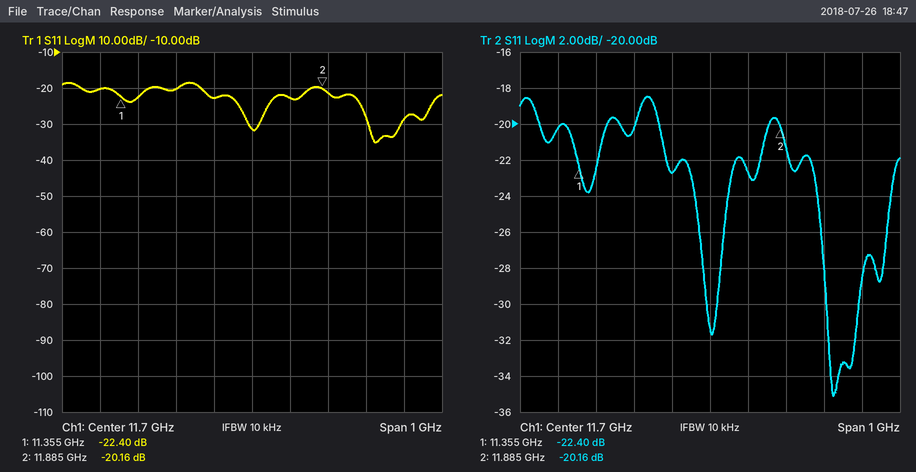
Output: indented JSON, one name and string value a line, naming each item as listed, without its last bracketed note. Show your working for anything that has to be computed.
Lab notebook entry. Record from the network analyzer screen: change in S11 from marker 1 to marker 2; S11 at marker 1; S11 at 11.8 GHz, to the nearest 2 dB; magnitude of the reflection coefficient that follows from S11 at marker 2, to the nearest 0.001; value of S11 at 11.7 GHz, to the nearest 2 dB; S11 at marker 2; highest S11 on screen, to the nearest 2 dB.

{
  "change in S11 from marker 1 to marker 2": "-20.16 − (-22.4) = 2.24 dB",
  "S11 at marker 1": "-22.40 dB",
  "S11 at 11.8 GHz, to the nearest 2 dB": "-22 dB",
  "magnitude of the reflection coefficient that follows from S11 at marker 2, to the nearest 0.001": "10^(-20.16/20) ≈ 0.098",
  "value of S11 at 11.7 GHz, to the nearest 2 dB": "-32 dB",
  "S11 at marker 2": "-20.16 dB",
  "highest S11 on screen, to the nearest 2 dB": "-18 dB"
}
